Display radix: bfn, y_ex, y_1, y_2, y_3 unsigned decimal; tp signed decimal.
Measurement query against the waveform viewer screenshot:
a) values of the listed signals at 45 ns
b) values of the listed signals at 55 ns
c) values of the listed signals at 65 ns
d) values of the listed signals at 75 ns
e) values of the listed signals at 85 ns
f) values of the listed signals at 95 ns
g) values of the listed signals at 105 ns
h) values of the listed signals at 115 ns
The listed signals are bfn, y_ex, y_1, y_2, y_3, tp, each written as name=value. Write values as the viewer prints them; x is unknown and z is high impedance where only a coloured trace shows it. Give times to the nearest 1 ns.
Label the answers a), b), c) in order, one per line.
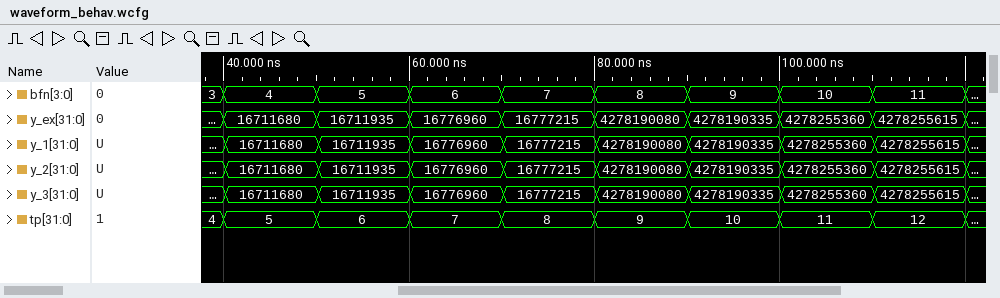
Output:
a) bfn=4, y_ex=16711680, y_1=16711680, y_2=16711680, y_3=16711680, tp=5
b) bfn=5, y_ex=16711935, y_1=16711935, y_2=16711935, y_3=16711935, tp=6
c) bfn=6, y_ex=16776960, y_1=16776960, y_2=16776960, y_3=16776960, tp=7
d) bfn=7, y_ex=16777215, y_1=16777215, y_2=16777215, y_3=16777215, tp=8
e) bfn=8, y_ex=4278190080, y_1=4278190080, y_2=4278190080, y_3=4278190080, tp=9
f) bfn=9, y_ex=4278190335, y_1=4278190335, y_2=4278190335, y_3=4278190335, tp=10
g) bfn=10, y_ex=4278255360, y_1=4278255360, y_2=4278255360, y_3=4278255360, tp=11
h) bfn=11, y_ex=4278255615, y_1=4278255615, y_2=4278255615, y_3=4278255615, tp=12
